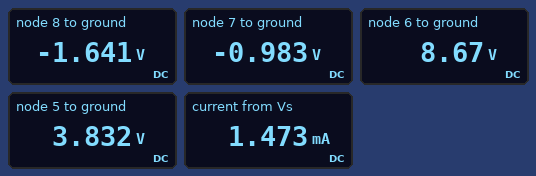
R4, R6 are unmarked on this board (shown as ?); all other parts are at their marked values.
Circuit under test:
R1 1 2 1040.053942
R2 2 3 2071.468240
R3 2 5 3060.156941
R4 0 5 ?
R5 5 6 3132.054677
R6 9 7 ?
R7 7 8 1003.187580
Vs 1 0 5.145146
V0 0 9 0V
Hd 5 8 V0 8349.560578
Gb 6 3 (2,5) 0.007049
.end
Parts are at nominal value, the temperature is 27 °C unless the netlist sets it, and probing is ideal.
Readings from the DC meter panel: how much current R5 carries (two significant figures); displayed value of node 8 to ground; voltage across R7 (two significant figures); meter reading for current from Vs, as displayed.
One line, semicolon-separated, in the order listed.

1.5 mA; -1.641 V; 660 mV; 1.473 mA
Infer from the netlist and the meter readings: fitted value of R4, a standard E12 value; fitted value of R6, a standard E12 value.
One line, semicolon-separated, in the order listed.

1.8 kΩ; 1.5 kΩ
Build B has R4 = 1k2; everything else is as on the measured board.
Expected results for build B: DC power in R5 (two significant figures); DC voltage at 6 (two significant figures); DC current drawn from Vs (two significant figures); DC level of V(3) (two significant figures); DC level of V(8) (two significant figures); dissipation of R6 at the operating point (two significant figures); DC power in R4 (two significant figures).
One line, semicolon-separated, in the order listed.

16 mW; 10 V; 2.1 mA; -1.7 V; -1.4 V; 460 µW; 8.7 mW
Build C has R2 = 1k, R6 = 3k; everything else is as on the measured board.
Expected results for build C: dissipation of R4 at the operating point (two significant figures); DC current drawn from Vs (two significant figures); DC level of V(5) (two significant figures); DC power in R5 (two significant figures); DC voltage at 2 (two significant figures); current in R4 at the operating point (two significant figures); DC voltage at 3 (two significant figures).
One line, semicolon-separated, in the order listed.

8.8 mW; 1.3 mA; 4.0 V; 5.8 mW; 3.8 V; 2.2 mA; 2.4 V
